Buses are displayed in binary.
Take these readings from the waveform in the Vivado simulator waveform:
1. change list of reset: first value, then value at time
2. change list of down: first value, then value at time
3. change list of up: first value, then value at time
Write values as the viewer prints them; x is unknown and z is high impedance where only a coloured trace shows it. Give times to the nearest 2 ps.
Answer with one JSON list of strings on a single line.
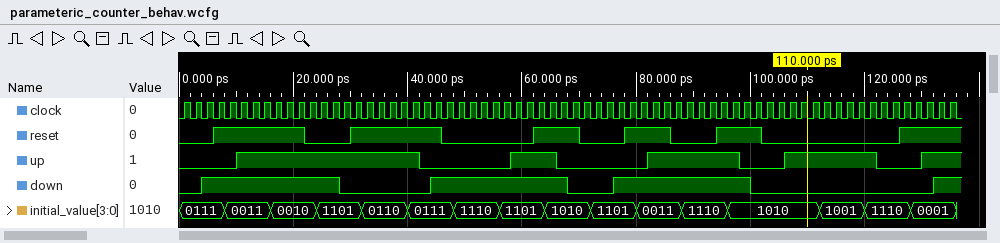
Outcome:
["0, 1 at 6 ps, 0 at 22 ps, 1 at 30 ps, 0 at 46 ps, 1 at 62 ps, 0 at 70 ps, 1 at 78 ps, 0 at 86 ps, 1 at 94 ps, 0 at 102 ps, 1 at 126 ps", "0, 1 at 4 ps, 0 at 28 ps, 1 at 44 ps, 0 at 68 ps, 1 at 76 ps, 0 at 100 ps, 1 at 132 ps", "0, 1 at 10 ps, 0 at 42 ps, 1 at 58 ps, 0 at 66 ps, 1 at 82 ps, 0 at 98 ps, 1 at 106 ps, 0 at 122 ps, 1 at 130 ps"]
